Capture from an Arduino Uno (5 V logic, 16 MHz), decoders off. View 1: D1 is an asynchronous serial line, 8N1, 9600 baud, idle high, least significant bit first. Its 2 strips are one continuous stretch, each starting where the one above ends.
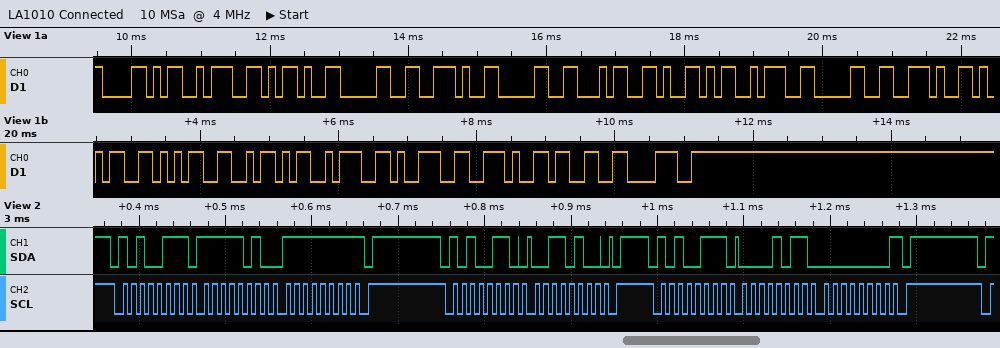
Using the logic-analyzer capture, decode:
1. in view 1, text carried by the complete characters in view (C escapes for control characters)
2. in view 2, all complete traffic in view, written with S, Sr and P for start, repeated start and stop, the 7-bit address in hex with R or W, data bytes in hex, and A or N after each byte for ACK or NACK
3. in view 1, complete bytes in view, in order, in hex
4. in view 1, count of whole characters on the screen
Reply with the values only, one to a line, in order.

"X:-0.04Y:0.55Z:9.38"
S 53R A FA A FF N P S 53W A 34 A P S 53R A 0B A 00 N P
0x58 0x3A 0x2D 0x30 0x2E 0x30 0x34 0x59 0x3A 0x30 0x2E 0x35 0x35 0x5A 0x3A 0x39 0x2E 0x33 0x38
19
